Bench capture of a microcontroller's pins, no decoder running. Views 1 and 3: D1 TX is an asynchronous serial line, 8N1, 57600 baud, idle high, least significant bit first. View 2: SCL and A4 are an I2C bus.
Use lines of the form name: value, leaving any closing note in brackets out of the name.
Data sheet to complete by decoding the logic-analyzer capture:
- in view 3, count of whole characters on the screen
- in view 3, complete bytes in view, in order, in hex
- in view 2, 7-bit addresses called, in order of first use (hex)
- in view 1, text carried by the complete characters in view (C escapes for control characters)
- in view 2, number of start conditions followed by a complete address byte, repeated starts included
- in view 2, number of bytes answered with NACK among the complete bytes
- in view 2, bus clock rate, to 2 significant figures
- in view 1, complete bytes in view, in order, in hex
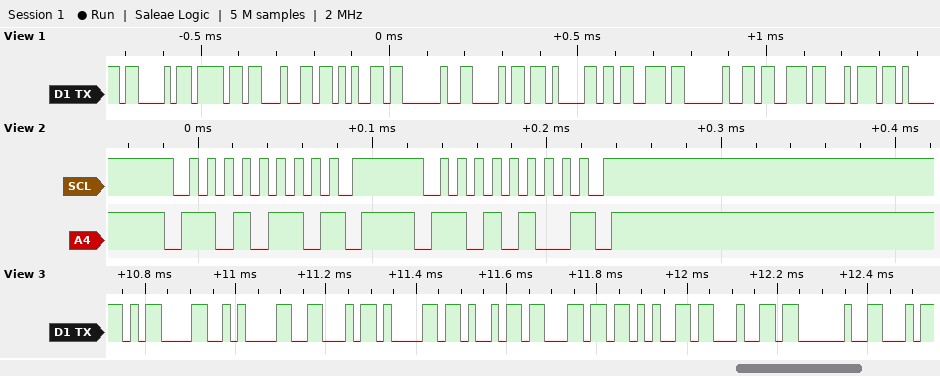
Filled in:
in view 3, count of whole characters on the screen: 9
in view 3, complete bytes in view, in order, in hex: 0D 0A 46 61 69 6C 65 64 20
in view 2, 7-bit addresses called, in order of first use: 0x6B 0x6A
in view 1, text carried by the complete characters in view: "Code has st"
in view 2, number of start conditions followed by a complete address byte, repeated starts included: 2
in view 2, number of bytes answered with NACK among the complete bytes: 2
in view 2, bus clock rate, to 2 significant figures: 100 kHz
in view 1, complete bytes in view, in order, in hex: 43 6F 64 65 20 68 61 73 20 73 74
